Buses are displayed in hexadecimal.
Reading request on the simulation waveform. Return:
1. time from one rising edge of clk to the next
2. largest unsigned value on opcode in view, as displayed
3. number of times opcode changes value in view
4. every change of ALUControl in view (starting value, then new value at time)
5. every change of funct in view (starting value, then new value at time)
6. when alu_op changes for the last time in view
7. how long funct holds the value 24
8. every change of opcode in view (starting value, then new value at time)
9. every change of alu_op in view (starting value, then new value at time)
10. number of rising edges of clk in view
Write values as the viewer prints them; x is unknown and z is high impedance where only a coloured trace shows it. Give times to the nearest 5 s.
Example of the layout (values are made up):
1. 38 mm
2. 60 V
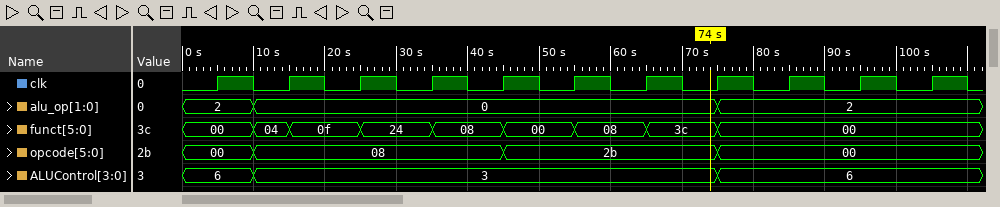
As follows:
1. 10 s
2. 2b
3. 3
4. 6, 3 at 10 s, 6 at 75 s
5. 00, 04 at 10 s, 0f at 15 s, 24 at 25 s, 08 at 35 s, 00 at 45 s, 08 at 55 s, 3c at 65 s, 00 at 75 s
6. 75 s
7. 10 s
8. 00, 08 at 10 s, 2b at 45 s, 00 at 75 s
9. 2, 0 at 10 s, 2 at 75 s
10. 11
